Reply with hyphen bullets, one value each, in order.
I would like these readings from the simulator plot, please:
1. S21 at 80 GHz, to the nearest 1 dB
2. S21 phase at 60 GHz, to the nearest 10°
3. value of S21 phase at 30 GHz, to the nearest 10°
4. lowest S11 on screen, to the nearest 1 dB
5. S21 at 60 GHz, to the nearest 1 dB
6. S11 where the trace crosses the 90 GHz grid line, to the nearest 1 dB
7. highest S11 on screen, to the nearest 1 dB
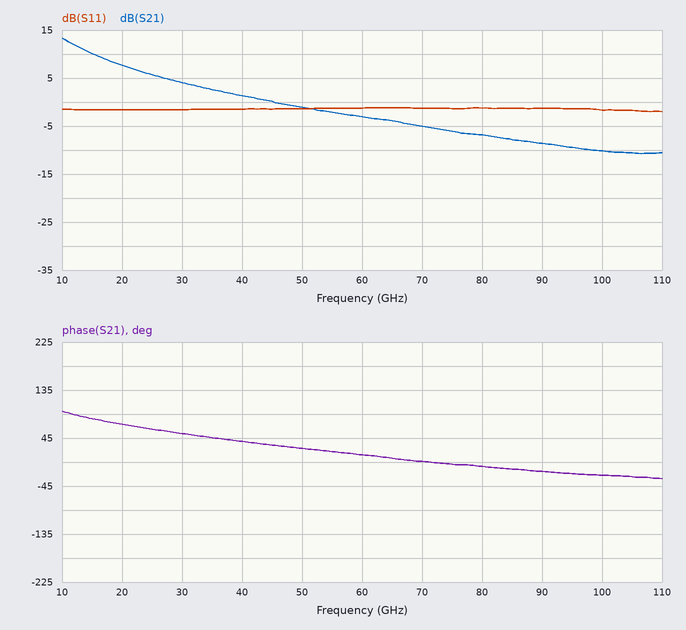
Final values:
- -7 dB
- 10°
- 50°
- -2 dB
- -3 dB
- -1 dB
- -1 dB
